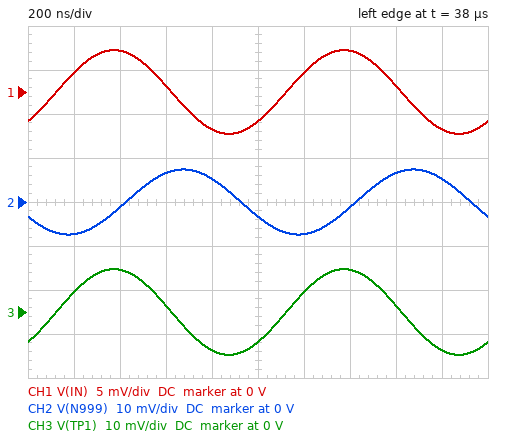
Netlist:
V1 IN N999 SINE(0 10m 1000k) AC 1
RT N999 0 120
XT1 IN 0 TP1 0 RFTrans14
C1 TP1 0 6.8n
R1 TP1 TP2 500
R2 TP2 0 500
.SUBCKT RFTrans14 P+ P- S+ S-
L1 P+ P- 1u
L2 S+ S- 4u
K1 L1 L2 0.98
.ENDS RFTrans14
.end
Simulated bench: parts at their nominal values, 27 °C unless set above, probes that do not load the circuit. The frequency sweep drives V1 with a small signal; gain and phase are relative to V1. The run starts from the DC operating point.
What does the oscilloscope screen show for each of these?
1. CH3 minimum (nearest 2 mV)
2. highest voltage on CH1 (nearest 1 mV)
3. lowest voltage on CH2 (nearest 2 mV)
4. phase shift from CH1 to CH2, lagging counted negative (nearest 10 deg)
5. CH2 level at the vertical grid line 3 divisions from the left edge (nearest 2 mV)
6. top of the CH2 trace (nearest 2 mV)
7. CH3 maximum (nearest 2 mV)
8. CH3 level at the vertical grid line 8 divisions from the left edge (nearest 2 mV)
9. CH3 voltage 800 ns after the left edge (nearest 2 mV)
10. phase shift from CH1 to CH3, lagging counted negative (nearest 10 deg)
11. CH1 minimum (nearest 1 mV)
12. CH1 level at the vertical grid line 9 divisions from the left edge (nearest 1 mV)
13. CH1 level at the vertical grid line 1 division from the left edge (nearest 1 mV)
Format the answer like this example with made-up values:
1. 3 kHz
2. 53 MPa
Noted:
1. -10 mV
2. 5 mV
3. -8 mV
4. -110 deg
5. 6 mV
6. 8 mV
7. 10 mV
8. 2 mV
9. -8 mV
10. 0 deg
11. -5 mV
12. -4 mV
13. 2 mV
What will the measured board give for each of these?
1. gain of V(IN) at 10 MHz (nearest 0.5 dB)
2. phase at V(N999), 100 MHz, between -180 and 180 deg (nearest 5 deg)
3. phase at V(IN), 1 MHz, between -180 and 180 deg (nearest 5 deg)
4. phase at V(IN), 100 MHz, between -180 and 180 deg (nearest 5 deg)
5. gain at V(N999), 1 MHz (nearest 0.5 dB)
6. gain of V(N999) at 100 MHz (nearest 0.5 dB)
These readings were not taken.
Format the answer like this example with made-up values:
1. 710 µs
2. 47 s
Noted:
1. -36.0 dB
2. 170 deg
3. -45 deg
4. 80 deg
5. -2.5 dB
6. 0 dB
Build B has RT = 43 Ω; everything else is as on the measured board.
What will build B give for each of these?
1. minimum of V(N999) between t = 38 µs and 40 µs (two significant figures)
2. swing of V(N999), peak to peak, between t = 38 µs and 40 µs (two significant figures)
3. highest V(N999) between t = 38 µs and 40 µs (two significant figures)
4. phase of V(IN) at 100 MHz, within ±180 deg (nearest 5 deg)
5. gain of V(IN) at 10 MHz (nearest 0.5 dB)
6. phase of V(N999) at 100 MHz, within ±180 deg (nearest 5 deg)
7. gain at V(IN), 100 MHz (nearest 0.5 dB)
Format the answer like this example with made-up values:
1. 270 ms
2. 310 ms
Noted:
1. -4.3 mV
2. 8.6 mV
3. 4.3 mV
4. 60 deg
5. -27.0 dB
6. 150 deg
7. -6.0 dB
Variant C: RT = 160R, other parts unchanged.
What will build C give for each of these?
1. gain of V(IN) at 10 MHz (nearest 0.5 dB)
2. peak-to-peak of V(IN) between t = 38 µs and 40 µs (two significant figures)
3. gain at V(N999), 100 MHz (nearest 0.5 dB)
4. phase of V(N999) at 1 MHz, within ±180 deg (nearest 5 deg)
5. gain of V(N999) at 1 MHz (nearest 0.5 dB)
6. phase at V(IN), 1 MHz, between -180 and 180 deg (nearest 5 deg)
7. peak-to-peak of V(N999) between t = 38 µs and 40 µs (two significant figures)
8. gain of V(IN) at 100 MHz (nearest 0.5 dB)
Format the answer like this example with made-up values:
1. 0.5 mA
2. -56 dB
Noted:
1. -38.5 dB
2. 7.8 mV
3. 0 dB
4. -160 deg
5. -2.0 dB
6. -50 deg
7. 16 mV
8. -16.5 dB
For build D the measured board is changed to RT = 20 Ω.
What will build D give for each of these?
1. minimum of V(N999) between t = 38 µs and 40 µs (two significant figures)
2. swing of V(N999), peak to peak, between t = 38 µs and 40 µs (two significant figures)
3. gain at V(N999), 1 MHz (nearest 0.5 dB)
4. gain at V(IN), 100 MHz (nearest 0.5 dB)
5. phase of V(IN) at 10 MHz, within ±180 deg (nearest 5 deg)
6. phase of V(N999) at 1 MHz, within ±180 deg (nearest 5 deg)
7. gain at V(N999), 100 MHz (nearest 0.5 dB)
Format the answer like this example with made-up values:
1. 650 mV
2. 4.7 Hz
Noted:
1. -2.3 mV
2. 4.7 mV
3. -12.5 dB
4. -2.0 dB
5. 85 deg
6. -120 deg
7. -4.0 dB
